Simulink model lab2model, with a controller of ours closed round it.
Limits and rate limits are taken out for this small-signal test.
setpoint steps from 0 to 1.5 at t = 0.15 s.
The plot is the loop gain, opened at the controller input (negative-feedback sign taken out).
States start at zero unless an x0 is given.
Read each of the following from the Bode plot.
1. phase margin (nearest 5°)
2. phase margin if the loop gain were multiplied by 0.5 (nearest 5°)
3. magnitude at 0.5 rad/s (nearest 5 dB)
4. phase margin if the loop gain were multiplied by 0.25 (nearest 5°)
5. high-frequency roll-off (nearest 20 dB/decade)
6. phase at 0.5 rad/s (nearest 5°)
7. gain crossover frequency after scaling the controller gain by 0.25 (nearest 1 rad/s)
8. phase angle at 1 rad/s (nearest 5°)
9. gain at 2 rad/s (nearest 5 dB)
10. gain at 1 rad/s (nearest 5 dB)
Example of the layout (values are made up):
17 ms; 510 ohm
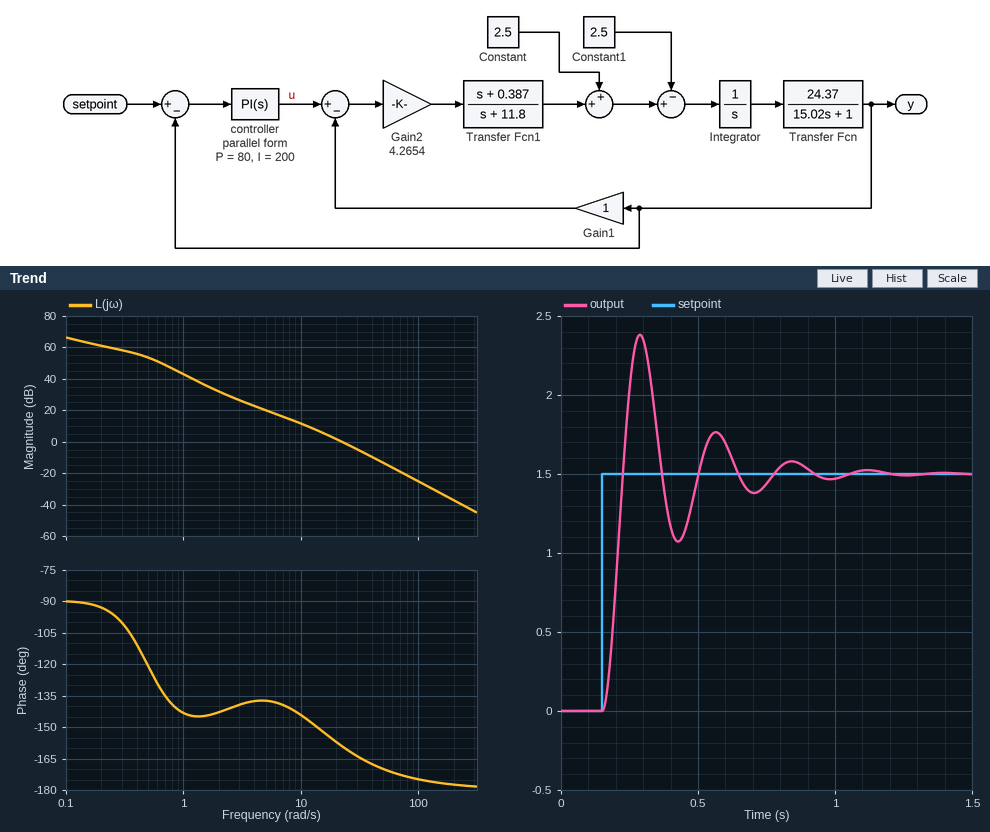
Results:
20°; 30°; 55 dB; 35°; -40 dB/decade; -120°; 10 rad/s; -145°; 30 dB; 45 dB
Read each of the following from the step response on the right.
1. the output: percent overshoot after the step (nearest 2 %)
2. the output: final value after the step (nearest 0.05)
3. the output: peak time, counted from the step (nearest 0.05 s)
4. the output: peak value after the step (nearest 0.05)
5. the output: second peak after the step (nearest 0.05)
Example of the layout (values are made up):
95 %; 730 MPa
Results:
58 %; 1.50; 0.15 s; 2.40; 1.75
